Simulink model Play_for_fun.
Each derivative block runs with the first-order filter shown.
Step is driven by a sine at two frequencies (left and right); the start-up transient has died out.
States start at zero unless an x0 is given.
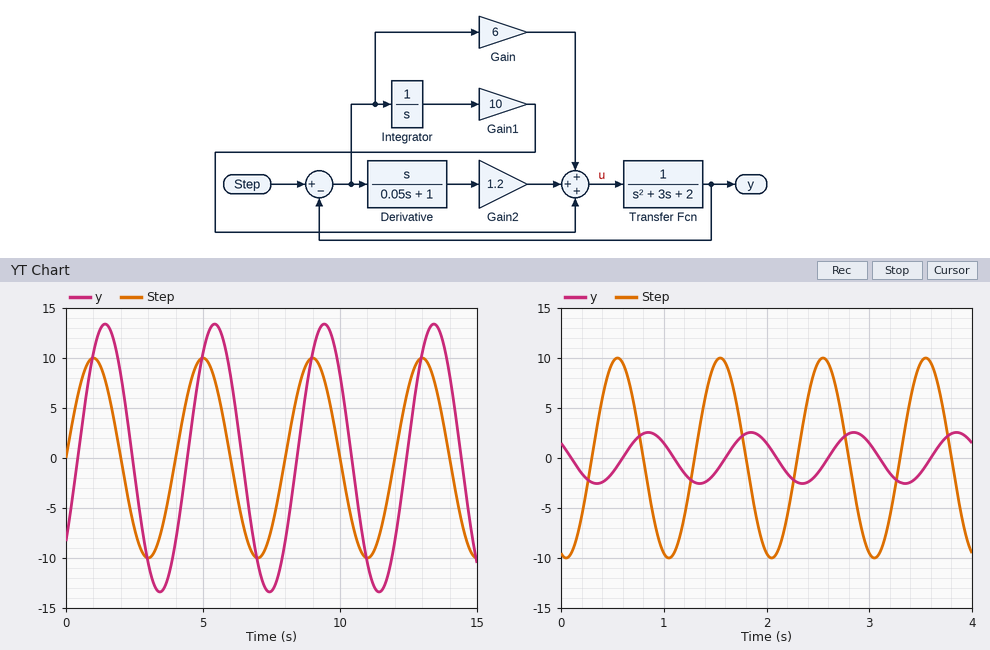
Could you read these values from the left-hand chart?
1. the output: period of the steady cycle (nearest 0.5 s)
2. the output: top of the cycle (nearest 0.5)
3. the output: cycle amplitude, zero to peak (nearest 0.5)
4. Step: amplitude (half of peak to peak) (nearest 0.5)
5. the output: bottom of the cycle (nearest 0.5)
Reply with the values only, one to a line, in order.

4.0 s
13.5
13.5
10.0
-13.5
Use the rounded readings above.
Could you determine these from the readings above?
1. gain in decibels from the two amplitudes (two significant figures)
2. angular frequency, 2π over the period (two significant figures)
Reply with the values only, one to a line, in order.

2.6 dB
1.6 rad/s
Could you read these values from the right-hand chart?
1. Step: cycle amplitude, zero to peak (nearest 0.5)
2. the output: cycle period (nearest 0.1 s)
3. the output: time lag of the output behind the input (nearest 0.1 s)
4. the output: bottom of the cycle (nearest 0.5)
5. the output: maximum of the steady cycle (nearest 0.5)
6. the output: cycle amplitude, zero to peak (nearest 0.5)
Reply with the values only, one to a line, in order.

10.0
1.0 s
0.3 s
-2.5
2.5
2.5
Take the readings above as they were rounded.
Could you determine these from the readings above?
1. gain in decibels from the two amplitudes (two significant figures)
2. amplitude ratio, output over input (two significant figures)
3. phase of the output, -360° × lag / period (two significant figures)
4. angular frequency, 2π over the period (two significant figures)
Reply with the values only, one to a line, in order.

-12 dB
0.25
-110°
6.3 rad/s
